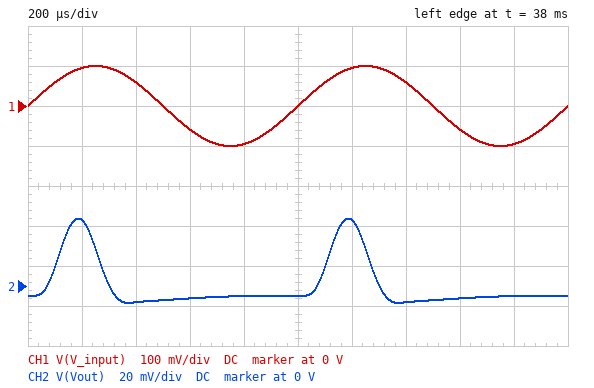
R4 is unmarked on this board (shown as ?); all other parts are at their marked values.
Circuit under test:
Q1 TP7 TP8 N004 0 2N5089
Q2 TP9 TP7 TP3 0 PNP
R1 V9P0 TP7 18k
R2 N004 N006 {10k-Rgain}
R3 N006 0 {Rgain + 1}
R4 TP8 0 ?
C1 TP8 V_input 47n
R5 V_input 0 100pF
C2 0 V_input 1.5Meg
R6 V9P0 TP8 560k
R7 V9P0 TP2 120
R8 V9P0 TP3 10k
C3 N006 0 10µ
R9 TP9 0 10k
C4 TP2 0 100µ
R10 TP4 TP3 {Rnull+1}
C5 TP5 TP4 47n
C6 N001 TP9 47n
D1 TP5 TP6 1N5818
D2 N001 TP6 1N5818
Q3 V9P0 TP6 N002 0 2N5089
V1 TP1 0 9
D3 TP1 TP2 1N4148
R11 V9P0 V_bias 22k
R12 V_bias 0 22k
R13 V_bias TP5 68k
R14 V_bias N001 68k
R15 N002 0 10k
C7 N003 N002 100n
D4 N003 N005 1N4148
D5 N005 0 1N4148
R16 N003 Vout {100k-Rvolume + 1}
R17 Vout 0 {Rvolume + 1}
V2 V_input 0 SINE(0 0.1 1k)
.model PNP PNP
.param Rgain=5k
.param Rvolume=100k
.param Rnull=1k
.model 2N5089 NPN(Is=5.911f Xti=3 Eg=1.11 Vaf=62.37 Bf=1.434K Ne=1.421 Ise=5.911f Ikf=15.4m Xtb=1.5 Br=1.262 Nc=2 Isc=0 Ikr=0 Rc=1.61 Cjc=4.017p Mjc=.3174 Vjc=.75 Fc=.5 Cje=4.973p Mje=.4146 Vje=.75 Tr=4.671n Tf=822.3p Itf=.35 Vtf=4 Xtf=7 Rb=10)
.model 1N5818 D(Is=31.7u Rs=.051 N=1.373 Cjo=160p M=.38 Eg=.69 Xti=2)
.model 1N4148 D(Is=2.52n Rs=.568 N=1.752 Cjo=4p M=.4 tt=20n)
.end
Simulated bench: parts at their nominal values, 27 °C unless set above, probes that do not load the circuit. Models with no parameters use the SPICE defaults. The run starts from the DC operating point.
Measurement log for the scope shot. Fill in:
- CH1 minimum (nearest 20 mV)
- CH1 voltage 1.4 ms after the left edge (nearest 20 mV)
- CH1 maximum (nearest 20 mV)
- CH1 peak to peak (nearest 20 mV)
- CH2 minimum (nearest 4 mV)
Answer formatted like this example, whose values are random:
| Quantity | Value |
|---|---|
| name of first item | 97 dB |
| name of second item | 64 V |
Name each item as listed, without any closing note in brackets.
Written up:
| Quantity | Value |
|---|---|
| CH1 minimum | -100 mV |
| CH1 voltage 1.4 ms after the left edge | 60 mV |
| CH1 maximum | 100 mV |
| CH1 peak to peak | 200 mV |
| CH2 minimum | -8 mV |
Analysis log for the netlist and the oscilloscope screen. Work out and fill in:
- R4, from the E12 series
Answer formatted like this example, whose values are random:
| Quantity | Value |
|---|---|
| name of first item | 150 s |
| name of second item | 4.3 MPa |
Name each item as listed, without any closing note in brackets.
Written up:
| Quantity | Value |
|---|---|
| R4, from the E12 series | 68 kΩ |
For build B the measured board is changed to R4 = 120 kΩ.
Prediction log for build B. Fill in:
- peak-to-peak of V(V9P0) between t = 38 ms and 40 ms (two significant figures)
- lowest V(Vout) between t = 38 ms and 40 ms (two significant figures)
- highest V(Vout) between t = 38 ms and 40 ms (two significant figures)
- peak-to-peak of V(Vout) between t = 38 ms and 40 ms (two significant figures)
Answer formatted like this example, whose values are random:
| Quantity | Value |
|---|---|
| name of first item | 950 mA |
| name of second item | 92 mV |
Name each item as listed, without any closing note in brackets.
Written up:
| Quantity | Value |
|---|---|
| peak-to-peak of V(V9P0) between t = 38 ms and 40 ms | 13 mV |
| lowest V(Vout) between t = 38 ms and 40 ms | -120 mV |
| highest V(Vout) between t = 38 ms and 40 ms | 120 mV |
| peak-to-peak of V(Vout) between t = 38 ms and 40 ms | 240 mV |
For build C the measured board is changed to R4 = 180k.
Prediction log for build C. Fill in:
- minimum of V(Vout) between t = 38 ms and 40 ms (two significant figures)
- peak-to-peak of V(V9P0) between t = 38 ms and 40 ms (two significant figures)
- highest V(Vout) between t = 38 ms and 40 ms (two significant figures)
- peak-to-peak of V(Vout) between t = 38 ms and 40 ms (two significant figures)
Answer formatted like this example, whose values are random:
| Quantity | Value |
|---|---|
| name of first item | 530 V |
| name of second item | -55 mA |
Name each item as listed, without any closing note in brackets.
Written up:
| Quantity | Value |
|---|---|
| minimum of V(Vout) between t = 38 ms and 40 ms | -140 mV |
| peak-to-peak of V(V9P0) between t = 38 ms and 40 ms | 13 mV |
| highest V(Vout) between t = 38 ms and 40 ms | 120 mV |
| peak-to-peak of V(Vout) between t = 38 ms and 40 ms | 250 mV |
